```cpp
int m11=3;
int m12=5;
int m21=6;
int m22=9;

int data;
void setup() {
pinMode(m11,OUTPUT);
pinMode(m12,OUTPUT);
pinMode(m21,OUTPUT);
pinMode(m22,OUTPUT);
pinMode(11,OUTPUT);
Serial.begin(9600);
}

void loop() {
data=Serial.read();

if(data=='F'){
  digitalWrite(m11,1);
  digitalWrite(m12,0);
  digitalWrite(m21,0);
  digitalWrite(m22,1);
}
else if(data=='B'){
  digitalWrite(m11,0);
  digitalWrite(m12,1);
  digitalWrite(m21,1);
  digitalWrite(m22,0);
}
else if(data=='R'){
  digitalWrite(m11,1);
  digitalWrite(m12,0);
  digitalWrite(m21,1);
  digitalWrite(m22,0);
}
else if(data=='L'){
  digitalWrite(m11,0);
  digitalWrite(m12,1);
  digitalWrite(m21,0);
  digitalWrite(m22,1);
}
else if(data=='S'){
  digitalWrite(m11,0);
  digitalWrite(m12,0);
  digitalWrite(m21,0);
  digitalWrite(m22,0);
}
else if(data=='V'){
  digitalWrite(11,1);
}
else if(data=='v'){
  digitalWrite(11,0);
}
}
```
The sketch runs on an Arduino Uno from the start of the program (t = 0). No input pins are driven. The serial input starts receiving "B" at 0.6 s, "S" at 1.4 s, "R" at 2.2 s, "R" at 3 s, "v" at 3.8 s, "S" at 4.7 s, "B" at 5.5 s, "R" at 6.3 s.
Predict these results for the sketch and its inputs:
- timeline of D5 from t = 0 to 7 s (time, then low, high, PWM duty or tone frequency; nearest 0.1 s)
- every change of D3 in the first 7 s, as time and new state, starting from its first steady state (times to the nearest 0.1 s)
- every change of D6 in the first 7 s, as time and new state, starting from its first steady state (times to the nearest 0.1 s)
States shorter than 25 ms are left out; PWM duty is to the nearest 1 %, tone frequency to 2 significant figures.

0 s low; 0.6 s high; 1.4 s low; 5.5 s high; 6.3 s low
0 s low; 2.2 s high; 4.7 s low; 6.3 s high
0 s low; 0.6 s high; 1.4 s low; 2.2 s high; 4.7 s low; 5.5 s high
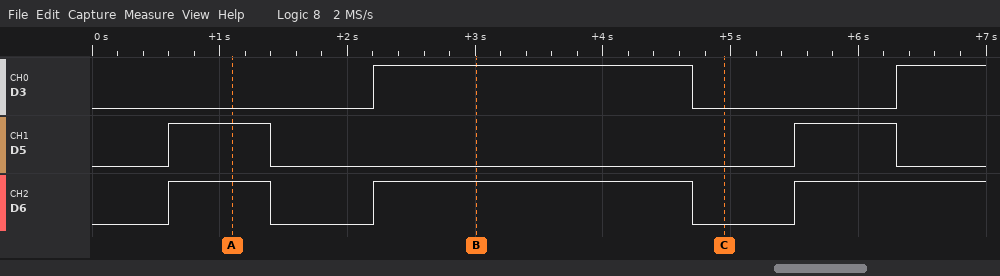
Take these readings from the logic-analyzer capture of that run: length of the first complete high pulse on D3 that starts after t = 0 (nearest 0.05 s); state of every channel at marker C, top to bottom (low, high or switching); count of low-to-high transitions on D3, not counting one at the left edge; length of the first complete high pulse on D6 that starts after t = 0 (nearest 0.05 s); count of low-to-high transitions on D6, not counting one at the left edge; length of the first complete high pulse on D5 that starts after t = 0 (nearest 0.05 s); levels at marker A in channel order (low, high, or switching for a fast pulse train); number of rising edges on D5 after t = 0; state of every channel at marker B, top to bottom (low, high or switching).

2.50 s
D3 low, D5 low, D6 low
2
0.80 s
3
0.80 s
D3 low, D5 high, D6 high
2
D3 high, D5 low, D6 high
